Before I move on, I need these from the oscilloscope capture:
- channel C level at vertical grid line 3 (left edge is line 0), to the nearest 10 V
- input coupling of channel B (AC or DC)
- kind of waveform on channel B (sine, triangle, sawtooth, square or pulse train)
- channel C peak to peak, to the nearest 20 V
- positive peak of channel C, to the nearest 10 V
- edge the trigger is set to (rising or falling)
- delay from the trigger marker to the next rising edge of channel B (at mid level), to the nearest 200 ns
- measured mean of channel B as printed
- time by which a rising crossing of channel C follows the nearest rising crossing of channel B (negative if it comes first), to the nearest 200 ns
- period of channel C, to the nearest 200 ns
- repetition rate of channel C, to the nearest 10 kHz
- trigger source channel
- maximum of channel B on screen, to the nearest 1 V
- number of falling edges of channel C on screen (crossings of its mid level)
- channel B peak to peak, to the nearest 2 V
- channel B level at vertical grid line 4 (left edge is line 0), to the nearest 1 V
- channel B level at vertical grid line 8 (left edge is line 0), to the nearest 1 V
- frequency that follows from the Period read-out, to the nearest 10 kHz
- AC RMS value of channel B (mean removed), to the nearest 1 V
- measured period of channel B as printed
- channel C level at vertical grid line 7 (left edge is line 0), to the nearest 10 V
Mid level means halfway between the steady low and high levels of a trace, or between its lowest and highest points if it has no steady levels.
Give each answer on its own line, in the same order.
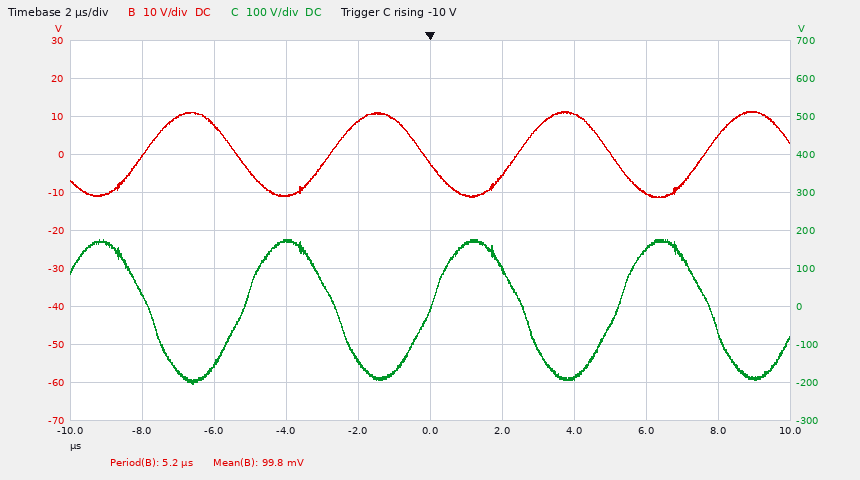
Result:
170 V
DC
sine
380 V
180 V
rising
2.4 µs
99.8 mV
-2.4 µs
5.2 µs
190 kHz
channel C
11 V
4
22 V
9 V
-10 V
190 kHz
8 V
5.2 µs
-190 V
